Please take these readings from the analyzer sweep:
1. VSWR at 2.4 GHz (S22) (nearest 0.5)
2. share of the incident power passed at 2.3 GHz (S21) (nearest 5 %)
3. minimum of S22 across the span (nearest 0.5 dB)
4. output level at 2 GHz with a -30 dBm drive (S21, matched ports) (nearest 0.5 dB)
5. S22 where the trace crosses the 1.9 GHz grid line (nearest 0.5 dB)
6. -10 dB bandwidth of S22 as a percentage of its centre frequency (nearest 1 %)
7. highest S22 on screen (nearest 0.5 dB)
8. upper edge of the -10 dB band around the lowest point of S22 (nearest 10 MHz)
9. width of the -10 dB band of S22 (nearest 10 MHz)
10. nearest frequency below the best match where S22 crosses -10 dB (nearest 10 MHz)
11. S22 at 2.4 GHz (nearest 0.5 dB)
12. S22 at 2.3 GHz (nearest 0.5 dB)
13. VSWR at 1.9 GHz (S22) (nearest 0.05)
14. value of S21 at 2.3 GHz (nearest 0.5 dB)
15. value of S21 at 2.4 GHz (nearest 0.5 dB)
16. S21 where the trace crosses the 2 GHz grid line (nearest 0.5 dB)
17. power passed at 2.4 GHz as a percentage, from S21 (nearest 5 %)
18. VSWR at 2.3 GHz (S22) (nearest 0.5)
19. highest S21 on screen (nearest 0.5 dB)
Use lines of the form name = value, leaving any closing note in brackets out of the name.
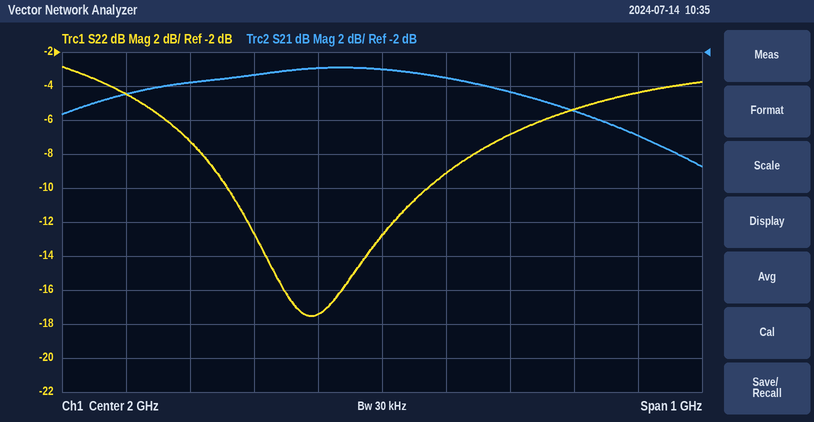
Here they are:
VSWR at 2.4 GHz (S22) = 4.0
share of the incident power passed at 2.3 GHz (S21) = 30 %
minimum of S22 across the span = -17.5 dB
output level at 2 GHz with a -30 dBm drive (S21, matched ports) = -33.0 dBm
S22 where the trace crosses the 1.9 GHz grid line = -17.5 dB
-10 dB bandwidth of S22 as a percentage of its centre frequency = 16 %
highest S22 on screen = -3.0 dB
upper edge of the -10 dB band around the lowest point of S22 = 2.07 GHz
width of the -10 dB band of S22 = 310 MHz
nearest frequency below the best match where S22 crosses -10 dB = 1.76 GHz
S22 at 2.4 GHz = -4.5 dB
S22 at 2.3 GHz = -5.5 dB
VSWR at 1.9 GHz (S22) = 1.30
value of S21 at 2.3 GHz = -5.5 dB
value of S21 at 2.4 GHz = -7.0 dB
S21 where the trace crosses the 2 GHz grid line = -3.0 dB
power passed at 2.4 GHz as a percentage, from S21 = 20 %
VSWR at 2.3 GHz (S22) = 3.5
highest S21 on screen = -3.0 dB
